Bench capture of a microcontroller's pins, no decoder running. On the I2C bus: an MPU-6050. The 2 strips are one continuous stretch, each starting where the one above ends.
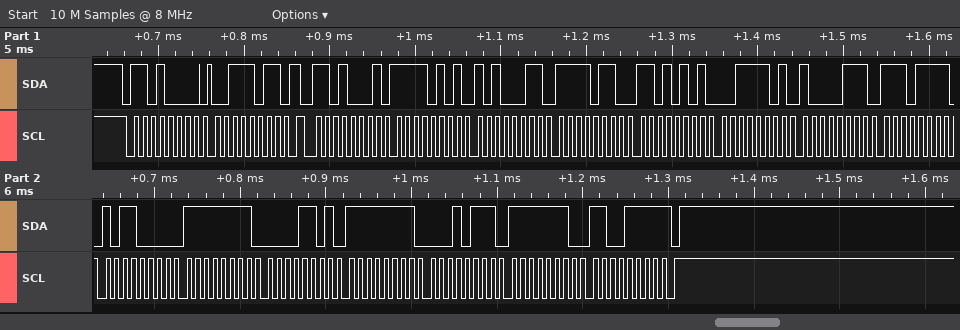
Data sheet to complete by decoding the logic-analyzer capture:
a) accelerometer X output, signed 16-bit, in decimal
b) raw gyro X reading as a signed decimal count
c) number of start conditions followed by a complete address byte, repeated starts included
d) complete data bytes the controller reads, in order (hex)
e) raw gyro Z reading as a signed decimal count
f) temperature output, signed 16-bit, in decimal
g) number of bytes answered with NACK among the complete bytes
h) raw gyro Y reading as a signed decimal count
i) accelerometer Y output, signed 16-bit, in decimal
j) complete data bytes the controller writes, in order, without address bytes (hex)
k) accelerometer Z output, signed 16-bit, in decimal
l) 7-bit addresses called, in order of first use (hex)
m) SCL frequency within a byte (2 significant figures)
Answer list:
-2653
-243
2
F5 A3 F6 D5 3D 87 EF B0 FF 0D FF 17 FE CF
-305
-4176
1
-233
-2347
3B
15751
0x68
100 kHz
